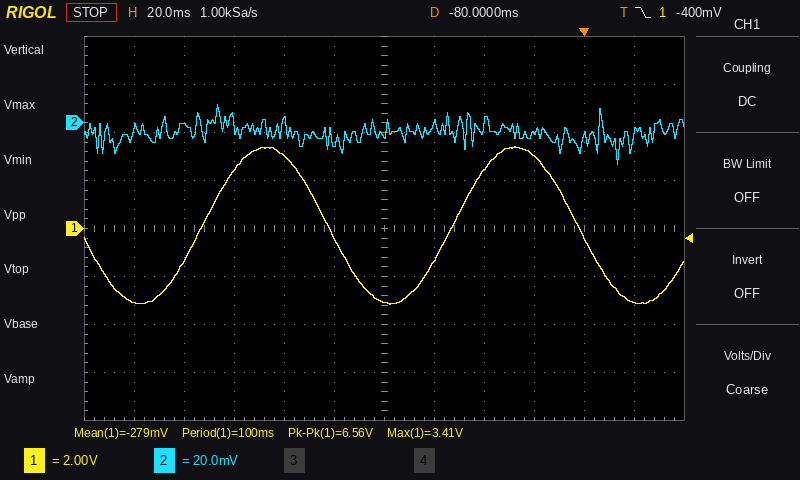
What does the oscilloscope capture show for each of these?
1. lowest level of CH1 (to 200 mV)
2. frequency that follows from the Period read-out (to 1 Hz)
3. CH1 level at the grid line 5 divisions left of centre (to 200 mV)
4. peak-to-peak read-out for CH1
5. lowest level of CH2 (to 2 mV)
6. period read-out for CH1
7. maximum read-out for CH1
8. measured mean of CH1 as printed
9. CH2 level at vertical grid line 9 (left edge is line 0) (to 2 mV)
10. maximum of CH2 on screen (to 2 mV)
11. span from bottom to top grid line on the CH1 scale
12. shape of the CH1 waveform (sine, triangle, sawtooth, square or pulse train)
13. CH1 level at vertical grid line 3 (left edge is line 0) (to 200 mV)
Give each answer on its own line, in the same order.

-3.2 V
10 Hz
-3.0 V
6.56 V
-18 mV
100 ms
3.41 V
-279 mV
-4 mV
8 mV
16 V
sine
2.4 V
